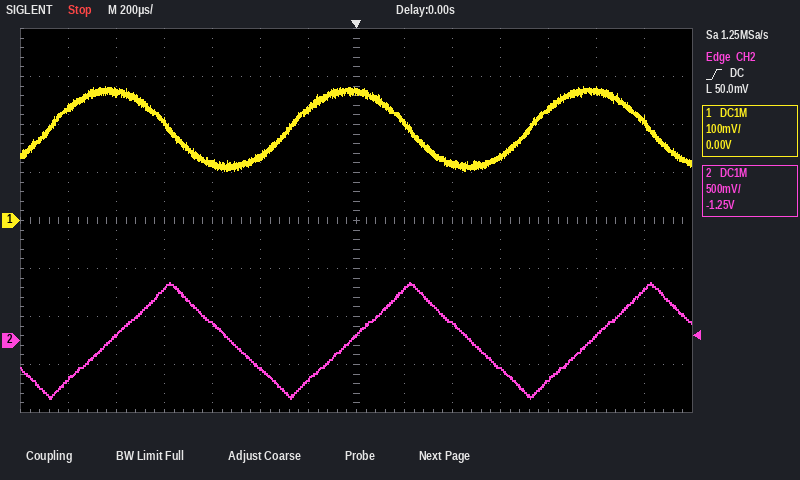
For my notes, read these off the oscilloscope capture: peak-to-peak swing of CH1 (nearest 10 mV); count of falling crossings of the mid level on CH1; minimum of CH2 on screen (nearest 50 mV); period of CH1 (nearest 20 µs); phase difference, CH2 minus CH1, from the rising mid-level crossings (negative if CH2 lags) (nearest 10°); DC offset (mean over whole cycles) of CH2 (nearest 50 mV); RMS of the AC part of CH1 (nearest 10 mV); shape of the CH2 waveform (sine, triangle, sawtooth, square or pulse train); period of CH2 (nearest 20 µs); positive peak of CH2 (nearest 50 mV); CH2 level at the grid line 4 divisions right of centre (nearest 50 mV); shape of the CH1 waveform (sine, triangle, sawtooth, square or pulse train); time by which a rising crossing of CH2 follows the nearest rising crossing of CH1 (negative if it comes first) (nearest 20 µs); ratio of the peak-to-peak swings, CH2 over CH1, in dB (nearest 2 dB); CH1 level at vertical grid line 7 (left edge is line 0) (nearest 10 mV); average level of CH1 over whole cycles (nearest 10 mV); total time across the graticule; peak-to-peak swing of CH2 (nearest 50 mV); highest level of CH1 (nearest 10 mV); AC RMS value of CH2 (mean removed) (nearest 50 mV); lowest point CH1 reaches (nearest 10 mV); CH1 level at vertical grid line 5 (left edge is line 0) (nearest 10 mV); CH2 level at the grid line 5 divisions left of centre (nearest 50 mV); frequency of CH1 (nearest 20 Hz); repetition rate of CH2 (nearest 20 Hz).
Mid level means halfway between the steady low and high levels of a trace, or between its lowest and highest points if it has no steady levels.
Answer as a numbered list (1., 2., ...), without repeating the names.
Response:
1. 180 mV
2. 3
3. -600 mV
4. 1.00 ms
5. -90°
6. 0 mV
7. 60 mV
8. triangle
9. 1.00 ms
10. 600 mV
11. -400 mV
12. sine
13. +260 µs
14. 16 dB
15. 270 mV
16. 190 mV
17. 2.8 ms
18. 1.20 V
19. 280 mV
20. 350 mV
21. 100 mV
22. 130 mV
23. 50 mV
24. 1.00 kHz
25. 1.00 kHz
